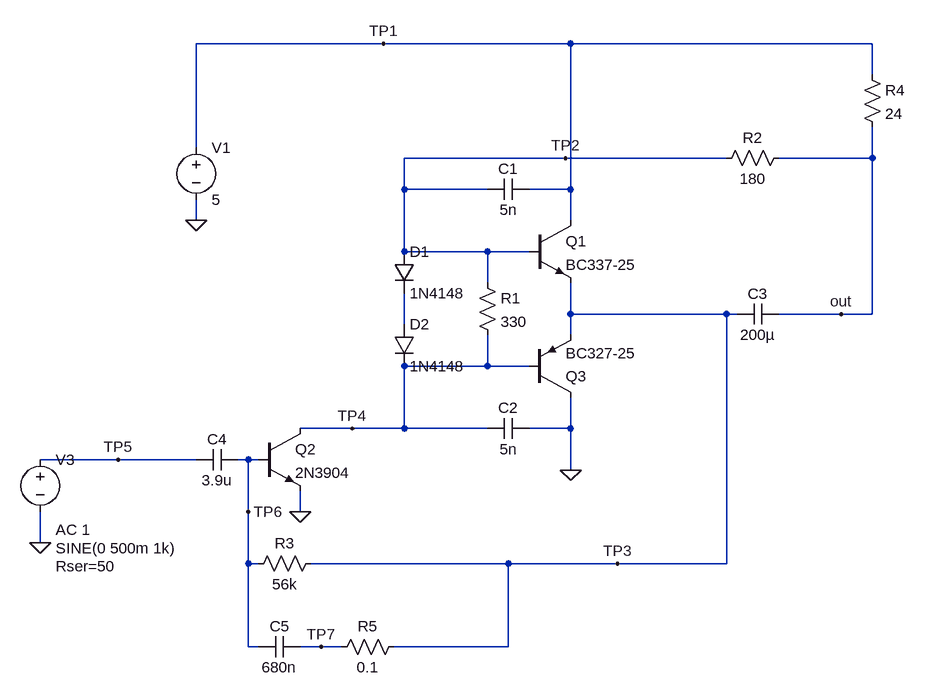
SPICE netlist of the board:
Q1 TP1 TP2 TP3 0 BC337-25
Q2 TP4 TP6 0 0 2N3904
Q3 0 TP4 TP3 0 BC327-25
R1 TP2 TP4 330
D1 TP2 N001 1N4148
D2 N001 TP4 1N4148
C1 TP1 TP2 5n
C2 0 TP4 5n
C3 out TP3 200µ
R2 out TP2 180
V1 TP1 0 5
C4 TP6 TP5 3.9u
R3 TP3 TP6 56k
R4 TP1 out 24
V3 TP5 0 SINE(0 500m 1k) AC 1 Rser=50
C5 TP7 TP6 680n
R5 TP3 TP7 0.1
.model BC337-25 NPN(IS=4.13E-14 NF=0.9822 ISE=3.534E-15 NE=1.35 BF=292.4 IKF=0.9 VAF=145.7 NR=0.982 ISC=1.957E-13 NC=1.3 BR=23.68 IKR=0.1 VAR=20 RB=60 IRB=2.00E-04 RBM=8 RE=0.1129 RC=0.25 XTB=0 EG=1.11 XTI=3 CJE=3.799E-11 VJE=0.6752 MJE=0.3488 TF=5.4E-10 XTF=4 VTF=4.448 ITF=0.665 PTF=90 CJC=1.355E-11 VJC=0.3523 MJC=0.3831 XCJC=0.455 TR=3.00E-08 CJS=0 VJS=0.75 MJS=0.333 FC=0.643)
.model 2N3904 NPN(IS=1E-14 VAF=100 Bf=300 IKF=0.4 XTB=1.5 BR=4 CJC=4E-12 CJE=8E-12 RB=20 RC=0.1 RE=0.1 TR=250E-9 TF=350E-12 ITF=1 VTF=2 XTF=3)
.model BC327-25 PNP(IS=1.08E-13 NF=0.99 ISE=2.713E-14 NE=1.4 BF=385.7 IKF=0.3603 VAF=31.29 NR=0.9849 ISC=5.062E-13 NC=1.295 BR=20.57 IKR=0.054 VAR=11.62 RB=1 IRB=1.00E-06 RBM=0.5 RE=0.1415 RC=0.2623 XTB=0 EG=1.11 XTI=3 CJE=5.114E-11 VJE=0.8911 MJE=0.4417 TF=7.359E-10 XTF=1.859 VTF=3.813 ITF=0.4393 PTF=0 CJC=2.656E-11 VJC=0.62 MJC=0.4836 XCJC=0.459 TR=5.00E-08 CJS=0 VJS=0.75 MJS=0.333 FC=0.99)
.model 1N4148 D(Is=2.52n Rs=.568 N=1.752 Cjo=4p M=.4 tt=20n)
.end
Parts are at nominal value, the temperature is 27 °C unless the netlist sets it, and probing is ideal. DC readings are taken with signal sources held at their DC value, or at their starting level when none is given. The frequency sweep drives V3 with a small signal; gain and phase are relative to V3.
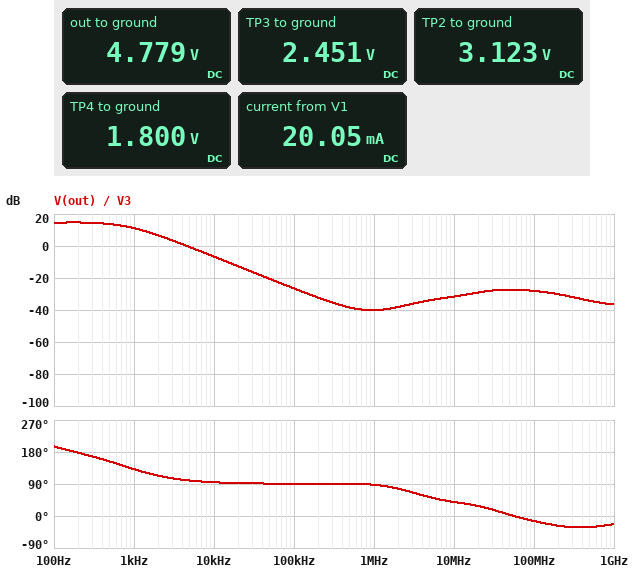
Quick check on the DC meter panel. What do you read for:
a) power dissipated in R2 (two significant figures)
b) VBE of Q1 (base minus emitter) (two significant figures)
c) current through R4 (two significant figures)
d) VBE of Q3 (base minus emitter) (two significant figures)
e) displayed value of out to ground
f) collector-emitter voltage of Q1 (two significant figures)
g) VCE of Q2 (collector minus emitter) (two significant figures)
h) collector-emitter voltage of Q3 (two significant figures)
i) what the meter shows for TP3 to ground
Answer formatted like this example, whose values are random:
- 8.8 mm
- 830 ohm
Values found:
- 15 mW
- 670 mV
- 9.2 mA
- -650 mV
- 4.779 V
- 2.5 V
- 1.8 V
- -2.5 V
- 2.451 V
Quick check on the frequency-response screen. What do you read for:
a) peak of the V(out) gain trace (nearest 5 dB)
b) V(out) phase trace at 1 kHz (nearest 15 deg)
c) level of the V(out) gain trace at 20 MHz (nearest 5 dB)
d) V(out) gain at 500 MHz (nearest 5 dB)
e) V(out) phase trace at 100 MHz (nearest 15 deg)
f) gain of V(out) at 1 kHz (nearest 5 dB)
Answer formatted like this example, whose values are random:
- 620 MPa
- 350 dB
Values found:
- 15 dB
- 135 deg
- -30 dB
- -35 dB
- -15 deg
- 10 dB
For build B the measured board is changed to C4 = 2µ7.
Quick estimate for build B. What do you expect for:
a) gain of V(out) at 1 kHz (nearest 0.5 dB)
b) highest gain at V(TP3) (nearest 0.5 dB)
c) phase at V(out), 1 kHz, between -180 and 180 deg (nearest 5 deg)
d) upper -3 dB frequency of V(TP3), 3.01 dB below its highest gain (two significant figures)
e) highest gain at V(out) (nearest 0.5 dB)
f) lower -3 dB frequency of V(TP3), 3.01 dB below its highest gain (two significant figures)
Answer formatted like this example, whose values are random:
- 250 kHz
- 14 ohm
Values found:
- 9.5 dB
- 12.0 dB
- 140 deg
- 1.2 kHz
- 11.5 dB
- 7.8 Hz
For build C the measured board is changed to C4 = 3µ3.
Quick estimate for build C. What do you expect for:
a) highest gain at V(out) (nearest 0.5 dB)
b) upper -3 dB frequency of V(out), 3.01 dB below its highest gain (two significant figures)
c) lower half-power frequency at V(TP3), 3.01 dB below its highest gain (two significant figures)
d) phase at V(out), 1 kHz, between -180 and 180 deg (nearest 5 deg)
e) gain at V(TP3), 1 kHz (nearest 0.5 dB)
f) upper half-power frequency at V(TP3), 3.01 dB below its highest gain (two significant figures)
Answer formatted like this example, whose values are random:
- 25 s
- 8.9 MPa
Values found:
- 13.5 dB
- 1.0 kHz
- 7.8 Hz
- 135 deg
- 10.5 dB
- 980 Hz
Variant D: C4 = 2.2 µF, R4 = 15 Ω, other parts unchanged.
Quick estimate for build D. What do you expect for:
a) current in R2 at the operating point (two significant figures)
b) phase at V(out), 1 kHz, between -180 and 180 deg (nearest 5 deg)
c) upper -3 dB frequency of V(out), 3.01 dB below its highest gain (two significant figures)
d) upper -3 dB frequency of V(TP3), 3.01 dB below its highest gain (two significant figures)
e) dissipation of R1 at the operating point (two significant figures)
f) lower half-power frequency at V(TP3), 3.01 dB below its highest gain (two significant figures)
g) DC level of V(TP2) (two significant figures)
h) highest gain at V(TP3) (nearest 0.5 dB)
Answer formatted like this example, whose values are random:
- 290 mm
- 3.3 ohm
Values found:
- 9.4 mA
- 150 deg
- 1.6 kHz
- 1.5 kHz
- 5.3 mW
- 8.1 Hz
- 3.2 V
- 10.0 dB
